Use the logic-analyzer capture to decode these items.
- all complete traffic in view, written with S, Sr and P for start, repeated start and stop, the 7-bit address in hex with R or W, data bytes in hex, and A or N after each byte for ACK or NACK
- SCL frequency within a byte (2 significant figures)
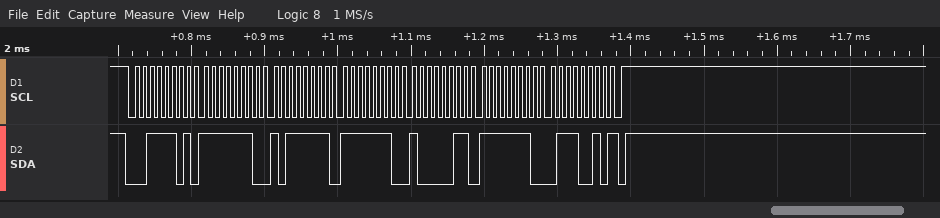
S 1ER A FE A BF A FE A 83 A FE A 72 N P
100 kHz
